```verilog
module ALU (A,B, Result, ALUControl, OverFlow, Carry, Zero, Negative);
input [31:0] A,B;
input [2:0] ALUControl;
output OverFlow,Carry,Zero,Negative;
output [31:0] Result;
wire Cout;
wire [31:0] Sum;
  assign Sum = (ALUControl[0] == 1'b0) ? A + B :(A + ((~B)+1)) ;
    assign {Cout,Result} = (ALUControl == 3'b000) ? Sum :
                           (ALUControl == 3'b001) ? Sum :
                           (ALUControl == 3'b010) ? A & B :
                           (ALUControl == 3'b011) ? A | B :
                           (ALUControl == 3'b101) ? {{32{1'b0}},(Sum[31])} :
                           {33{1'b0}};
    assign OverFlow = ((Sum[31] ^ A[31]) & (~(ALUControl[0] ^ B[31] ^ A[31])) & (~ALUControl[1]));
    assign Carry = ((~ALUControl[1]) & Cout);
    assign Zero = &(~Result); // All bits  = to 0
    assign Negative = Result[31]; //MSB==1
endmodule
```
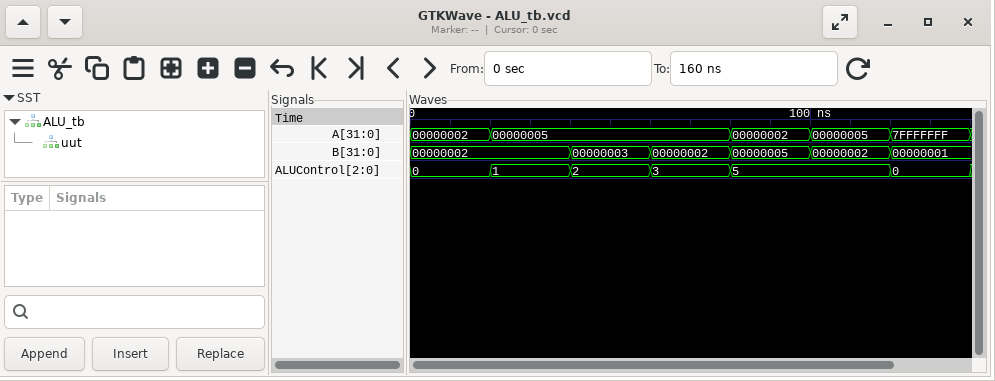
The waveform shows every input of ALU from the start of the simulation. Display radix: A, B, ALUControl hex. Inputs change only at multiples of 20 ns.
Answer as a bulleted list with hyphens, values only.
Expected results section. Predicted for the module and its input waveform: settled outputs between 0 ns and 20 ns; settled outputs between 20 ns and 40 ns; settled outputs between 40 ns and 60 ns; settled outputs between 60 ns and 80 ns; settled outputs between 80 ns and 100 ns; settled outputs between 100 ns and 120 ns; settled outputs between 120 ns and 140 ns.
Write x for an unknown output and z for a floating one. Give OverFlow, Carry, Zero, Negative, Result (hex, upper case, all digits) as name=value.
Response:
- OverFlow=0, Carry=0, Zero=0, Negative=0, Result=00000004
- OverFlow=0, Carry=0, Zero=0, Negative=0, Result=00000003
- OverFlow=0, Carry=0, Zero=0, Negative=0, Result=00000001
- OverFlow=0, Carry=0, Zero=0, Negative=0, Result=00000007
- OverFlow=0, Carry=0, Zero=0, Negative=0, Result=00000001
- OverFlow=0, Carry=0, Zero=1, Negative=0, Result=00000000
- OverFlow=1, Carry=0, Zero=0, Negative=1, Result=80000000
